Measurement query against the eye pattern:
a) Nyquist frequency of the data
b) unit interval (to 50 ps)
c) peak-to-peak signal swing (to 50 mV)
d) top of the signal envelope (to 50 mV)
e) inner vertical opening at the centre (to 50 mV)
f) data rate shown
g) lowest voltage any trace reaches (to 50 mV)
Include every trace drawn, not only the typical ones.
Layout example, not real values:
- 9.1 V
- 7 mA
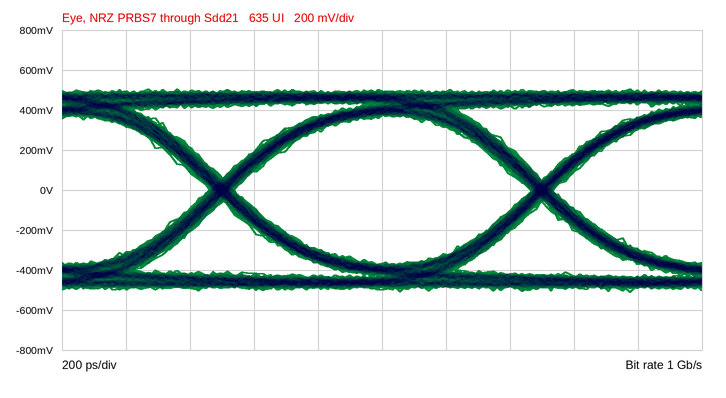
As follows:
- 500 MHz
- 1.00 ns
- 1.00 V
- 500 mV
- 750 mV
- 1 Gb/s
- -500 mV
